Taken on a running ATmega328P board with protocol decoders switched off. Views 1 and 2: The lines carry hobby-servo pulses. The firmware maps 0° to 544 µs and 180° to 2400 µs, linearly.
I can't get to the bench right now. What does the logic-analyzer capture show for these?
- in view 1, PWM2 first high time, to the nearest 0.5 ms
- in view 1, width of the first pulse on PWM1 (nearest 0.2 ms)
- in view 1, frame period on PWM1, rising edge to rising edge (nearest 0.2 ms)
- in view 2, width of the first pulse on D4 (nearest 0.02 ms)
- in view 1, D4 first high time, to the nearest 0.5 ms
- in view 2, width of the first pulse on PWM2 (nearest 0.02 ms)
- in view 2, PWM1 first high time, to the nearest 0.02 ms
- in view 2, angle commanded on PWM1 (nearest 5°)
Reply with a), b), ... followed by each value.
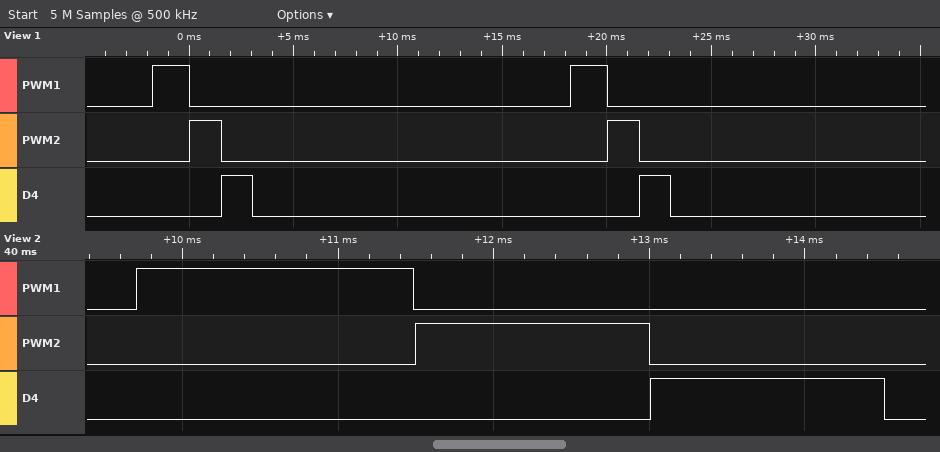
a) 1.5 ms
b) 1.8 ms
c) 20.0 ms
d) 1.50 ms
e) 1.5 ms
f) 1.50 ms
g) 1.78 ms
h) 120°
